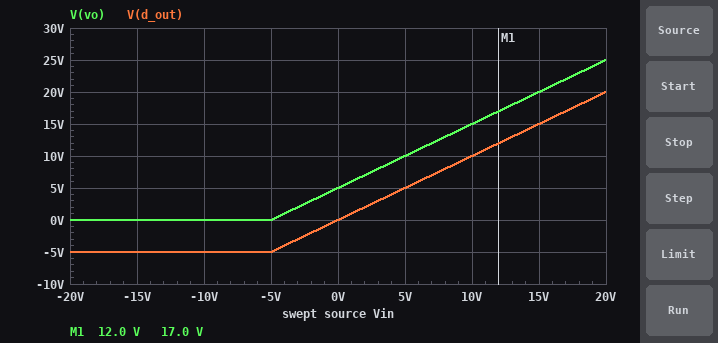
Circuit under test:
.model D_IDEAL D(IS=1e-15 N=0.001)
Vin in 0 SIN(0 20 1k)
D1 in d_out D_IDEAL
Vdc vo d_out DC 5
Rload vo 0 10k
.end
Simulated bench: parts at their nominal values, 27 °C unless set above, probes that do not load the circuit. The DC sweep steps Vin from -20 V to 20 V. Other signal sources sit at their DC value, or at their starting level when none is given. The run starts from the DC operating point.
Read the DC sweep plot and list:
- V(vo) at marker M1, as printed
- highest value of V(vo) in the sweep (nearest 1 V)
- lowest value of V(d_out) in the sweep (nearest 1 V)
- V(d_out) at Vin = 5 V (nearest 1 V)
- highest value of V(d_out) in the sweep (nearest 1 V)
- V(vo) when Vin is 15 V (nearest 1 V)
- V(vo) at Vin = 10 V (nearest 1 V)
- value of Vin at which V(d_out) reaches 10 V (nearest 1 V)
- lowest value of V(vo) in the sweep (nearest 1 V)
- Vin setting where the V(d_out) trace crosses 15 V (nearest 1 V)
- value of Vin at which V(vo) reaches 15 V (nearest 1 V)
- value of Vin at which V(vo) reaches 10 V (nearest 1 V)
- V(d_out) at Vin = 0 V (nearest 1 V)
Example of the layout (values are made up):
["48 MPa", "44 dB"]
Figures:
["17.0 V", "25 V", "-5 V", "5 V", "20 V", "20 V", "15 V", "10 V", "0 V", "15 V", "10 V", "5 V", "0 V"]
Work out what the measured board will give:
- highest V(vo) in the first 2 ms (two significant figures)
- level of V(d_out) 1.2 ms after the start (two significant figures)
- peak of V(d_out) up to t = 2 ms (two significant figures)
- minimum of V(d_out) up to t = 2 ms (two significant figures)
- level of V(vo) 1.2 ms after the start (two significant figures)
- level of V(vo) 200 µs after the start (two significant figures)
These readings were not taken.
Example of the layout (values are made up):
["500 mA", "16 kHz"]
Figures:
["25 V", "19 V", "20 V", "-5.0 V", "24 V", "24 V"]
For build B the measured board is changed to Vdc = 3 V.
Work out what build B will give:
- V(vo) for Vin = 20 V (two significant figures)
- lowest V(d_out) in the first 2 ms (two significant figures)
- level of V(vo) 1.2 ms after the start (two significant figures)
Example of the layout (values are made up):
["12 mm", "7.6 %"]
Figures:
["23 V", "-3.0 V", "22 V"]
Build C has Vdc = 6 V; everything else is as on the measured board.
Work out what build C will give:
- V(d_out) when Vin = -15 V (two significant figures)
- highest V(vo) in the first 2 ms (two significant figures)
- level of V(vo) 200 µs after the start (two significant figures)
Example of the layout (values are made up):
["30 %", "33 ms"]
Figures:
["-6.0 V", "26 V", "25 V"]
